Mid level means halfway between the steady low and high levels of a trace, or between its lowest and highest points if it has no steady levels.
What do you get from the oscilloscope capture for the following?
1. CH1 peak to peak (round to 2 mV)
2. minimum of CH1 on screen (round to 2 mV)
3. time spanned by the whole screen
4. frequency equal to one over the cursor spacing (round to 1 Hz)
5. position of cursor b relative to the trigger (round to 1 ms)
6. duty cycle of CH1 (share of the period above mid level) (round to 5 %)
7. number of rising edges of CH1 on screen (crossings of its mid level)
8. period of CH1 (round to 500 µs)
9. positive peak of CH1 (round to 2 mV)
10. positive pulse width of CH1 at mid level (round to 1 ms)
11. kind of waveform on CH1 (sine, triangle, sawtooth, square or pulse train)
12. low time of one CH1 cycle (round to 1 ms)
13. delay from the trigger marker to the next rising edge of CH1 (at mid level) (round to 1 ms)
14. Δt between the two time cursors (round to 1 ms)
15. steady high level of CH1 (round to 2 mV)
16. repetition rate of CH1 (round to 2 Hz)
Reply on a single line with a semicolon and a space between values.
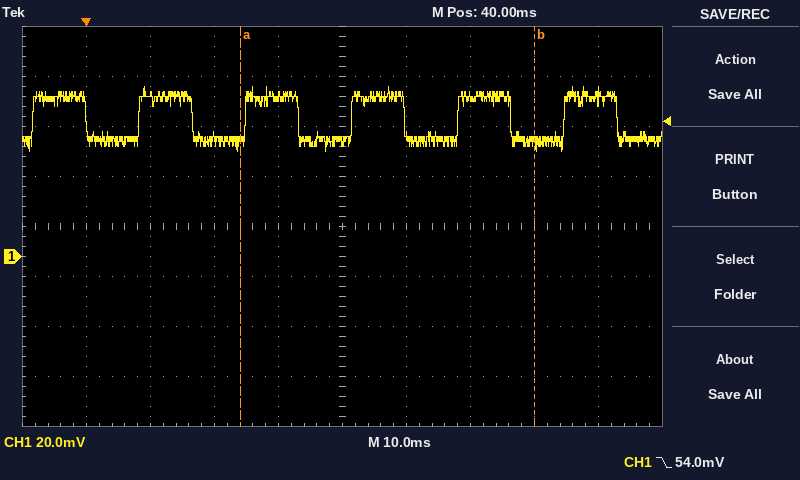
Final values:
26 mV; 42 mV; 100 ms; 22 Hz; +70 ms; 50 %; 6; 16.5 ms; 68 mV; 8 ms; square; 8 ms; 8 ms; 46 ms; 64 mV; 60 Hz
